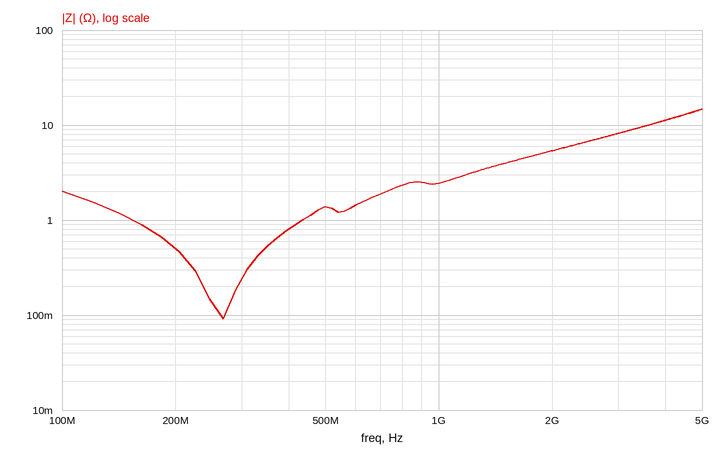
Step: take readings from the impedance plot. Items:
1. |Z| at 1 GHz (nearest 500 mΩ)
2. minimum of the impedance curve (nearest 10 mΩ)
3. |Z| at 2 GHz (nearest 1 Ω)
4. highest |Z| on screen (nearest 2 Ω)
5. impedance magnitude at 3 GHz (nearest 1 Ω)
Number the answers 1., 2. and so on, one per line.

1. 2.5 Ω
2. 90 mΩ
3. 5 Ω
4. 14 Ω
5. 8 Ω
